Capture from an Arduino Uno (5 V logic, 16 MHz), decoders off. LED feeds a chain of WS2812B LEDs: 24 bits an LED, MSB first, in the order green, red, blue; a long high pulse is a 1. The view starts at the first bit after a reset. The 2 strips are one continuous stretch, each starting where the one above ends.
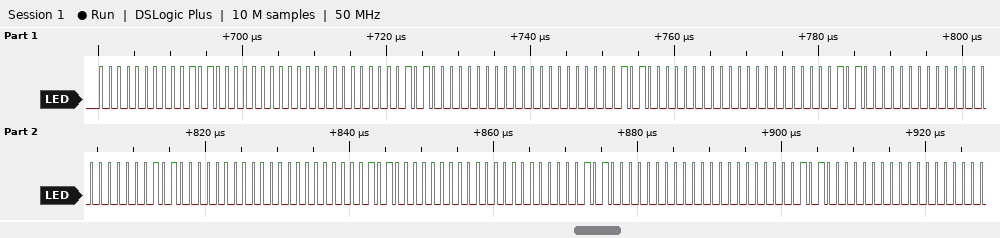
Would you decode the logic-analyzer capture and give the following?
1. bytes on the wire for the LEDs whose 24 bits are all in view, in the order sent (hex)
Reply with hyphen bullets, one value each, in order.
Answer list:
- 00 28 00 00 28 00 00 28 00 00 28 00 00 28 00 00 28 00 00 28 00 00 28 00
